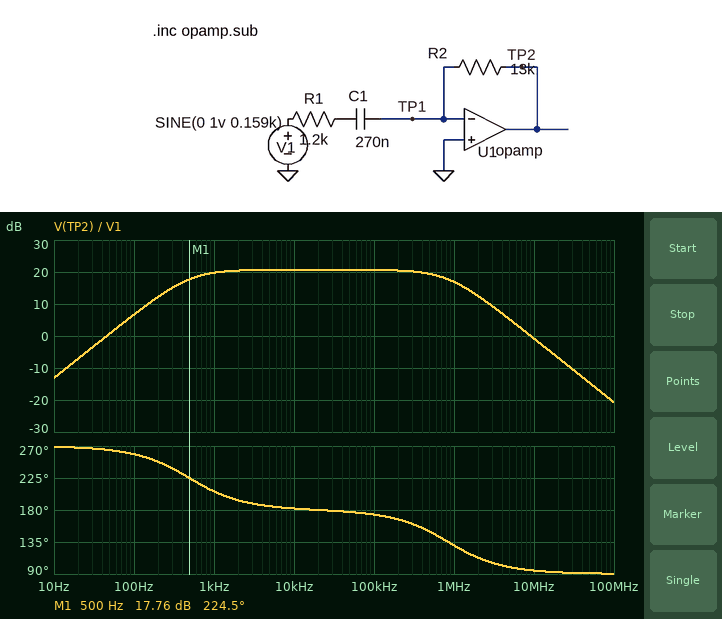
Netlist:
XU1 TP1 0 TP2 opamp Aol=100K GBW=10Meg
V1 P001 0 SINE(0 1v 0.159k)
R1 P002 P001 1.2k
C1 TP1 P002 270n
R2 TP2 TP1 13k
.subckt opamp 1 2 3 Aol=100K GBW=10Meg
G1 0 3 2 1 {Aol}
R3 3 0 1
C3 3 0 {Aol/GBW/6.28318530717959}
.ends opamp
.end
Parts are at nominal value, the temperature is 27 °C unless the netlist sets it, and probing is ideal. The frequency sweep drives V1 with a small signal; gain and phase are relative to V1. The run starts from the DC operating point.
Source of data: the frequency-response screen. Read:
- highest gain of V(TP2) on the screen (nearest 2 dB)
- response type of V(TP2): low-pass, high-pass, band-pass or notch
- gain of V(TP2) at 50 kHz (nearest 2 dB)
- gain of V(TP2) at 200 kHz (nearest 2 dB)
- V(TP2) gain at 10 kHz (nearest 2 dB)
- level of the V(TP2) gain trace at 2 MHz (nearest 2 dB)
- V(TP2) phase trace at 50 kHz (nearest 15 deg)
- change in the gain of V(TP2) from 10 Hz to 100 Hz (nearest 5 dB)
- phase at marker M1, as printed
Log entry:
20 dB
band-pass
20 dB
20 dB
20 dB
12 dB
180 deg
20 dB
224.5 deg
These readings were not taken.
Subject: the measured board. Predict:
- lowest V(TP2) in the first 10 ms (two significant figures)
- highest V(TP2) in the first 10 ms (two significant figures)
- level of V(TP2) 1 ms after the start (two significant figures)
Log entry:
-3.3 V
3.3 V
-2.4 V
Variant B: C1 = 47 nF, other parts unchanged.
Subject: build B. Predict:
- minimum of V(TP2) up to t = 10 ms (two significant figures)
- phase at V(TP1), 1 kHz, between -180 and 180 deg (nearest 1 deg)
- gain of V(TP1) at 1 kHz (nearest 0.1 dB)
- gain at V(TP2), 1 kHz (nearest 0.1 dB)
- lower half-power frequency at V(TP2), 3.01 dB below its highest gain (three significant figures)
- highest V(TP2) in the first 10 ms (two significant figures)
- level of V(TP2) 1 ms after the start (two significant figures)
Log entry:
-610 mV
155 deg
-68.8 dB
11.2 dB
2.81 kHz
610 mV
-360 mV
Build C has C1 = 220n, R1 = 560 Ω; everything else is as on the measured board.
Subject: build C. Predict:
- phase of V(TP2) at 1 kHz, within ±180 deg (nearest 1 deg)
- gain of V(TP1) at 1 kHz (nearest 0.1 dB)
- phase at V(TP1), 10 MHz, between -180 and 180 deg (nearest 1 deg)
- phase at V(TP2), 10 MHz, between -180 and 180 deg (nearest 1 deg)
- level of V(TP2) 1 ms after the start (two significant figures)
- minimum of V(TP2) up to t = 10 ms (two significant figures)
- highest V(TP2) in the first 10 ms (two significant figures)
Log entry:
-128 deg
-56.9 dB
2 deg
92 deg
-1.8 V
-2.8 V
2.8 V
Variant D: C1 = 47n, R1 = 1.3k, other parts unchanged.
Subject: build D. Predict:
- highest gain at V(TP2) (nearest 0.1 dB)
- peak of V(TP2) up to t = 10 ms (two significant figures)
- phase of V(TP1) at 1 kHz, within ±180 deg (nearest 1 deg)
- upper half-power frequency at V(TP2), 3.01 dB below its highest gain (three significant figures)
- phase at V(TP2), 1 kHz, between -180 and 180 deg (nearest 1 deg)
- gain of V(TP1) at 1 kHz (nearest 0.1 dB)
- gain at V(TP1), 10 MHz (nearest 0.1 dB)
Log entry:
20.0 dB
610 mV
153 deg
912 kHz
-111 deg
-68.9 dB
-0.9 dB
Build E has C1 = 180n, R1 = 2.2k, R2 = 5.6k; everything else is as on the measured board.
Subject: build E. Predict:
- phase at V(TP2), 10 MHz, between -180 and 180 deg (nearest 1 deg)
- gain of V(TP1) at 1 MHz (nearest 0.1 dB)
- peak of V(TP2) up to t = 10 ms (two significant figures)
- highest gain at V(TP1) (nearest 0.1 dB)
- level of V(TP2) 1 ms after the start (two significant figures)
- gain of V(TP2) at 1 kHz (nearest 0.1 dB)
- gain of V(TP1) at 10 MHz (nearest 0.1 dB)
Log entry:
106 deg
-12.4 dB
940 mV
-2.9 dB
-690 mV
7.5 dB
-3.2 dB
